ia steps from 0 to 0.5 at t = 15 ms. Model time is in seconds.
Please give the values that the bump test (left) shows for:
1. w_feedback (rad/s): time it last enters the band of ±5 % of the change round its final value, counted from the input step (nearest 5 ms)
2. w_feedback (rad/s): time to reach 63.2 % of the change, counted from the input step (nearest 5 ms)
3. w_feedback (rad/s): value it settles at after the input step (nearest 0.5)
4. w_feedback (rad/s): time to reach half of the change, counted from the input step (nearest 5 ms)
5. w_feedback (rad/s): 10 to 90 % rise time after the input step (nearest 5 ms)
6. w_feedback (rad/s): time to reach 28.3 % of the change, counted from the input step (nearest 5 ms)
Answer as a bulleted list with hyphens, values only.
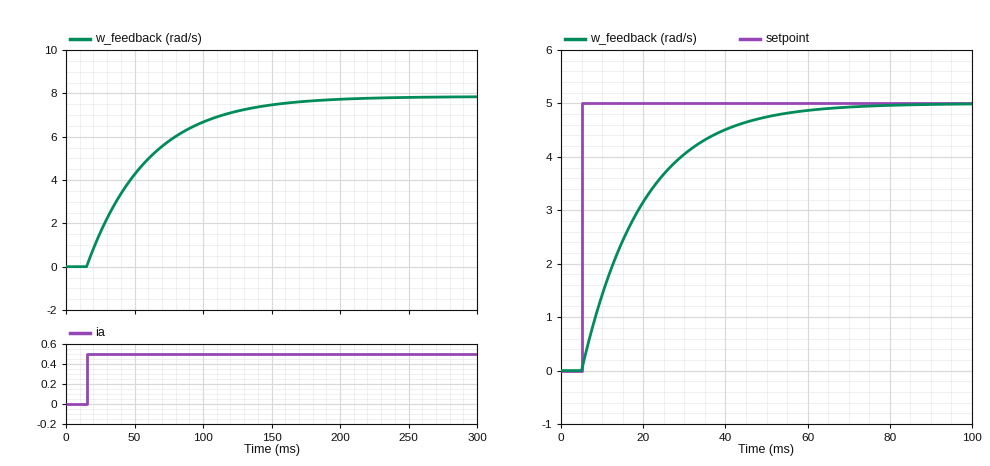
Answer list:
- 135 ms
- 45 ms
- 8.0
- 30 ms
- 100 ms
- 15 ms
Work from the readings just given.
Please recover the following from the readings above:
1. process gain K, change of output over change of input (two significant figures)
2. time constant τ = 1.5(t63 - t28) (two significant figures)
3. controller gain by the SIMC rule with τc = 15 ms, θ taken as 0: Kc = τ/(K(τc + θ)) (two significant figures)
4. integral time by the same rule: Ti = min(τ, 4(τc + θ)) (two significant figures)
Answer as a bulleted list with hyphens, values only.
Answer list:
- 16
- 45 ms
- 0.19
- 45 ms
